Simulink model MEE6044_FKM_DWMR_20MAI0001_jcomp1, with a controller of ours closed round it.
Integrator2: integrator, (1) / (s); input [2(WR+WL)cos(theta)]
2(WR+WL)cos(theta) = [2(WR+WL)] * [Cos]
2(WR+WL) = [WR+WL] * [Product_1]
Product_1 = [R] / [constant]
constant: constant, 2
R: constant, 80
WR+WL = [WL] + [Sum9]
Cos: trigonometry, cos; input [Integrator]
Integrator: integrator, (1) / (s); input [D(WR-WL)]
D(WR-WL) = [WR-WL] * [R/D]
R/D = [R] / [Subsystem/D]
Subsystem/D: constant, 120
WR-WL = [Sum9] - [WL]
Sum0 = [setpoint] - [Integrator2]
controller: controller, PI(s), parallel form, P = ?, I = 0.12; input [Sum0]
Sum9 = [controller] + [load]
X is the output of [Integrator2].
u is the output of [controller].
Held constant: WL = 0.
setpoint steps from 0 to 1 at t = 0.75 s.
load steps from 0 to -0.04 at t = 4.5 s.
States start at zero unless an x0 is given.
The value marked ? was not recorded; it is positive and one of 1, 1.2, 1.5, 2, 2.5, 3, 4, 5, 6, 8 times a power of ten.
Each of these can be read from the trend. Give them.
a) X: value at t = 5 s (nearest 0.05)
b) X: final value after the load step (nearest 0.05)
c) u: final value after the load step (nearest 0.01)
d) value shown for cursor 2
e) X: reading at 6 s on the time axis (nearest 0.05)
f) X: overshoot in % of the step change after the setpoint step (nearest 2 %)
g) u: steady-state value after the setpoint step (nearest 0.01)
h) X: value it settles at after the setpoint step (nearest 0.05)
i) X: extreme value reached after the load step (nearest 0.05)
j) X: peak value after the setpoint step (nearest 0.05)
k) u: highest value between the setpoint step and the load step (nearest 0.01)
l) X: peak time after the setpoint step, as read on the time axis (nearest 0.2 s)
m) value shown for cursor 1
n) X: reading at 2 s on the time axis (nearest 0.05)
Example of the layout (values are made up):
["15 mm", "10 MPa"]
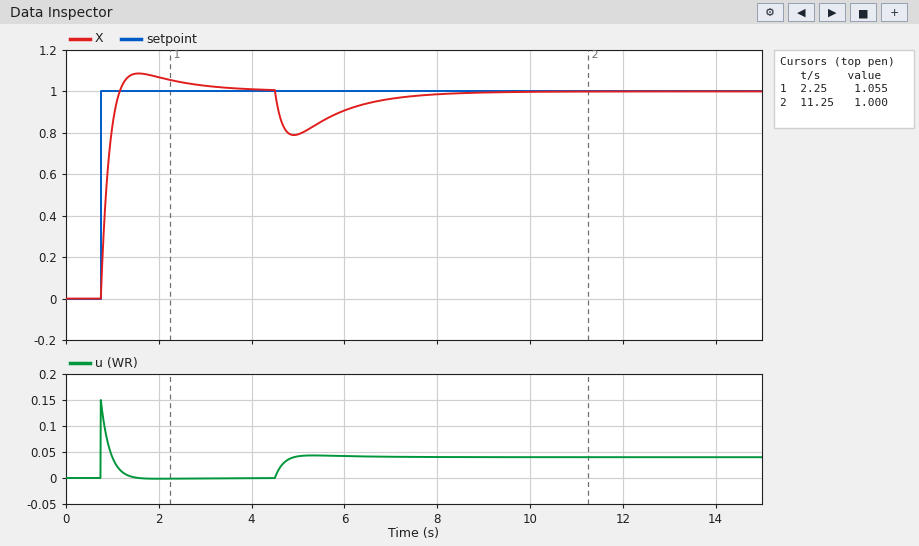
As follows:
["0.80", "1.00", "0.04", "1.000", "0.90", "8 %", "0.00", "1.00", "0.80", "1.10", "0.15", "1.6 s", "1.055", "1.05"]
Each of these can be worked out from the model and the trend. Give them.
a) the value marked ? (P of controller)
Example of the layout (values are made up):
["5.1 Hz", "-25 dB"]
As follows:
["0.15"]
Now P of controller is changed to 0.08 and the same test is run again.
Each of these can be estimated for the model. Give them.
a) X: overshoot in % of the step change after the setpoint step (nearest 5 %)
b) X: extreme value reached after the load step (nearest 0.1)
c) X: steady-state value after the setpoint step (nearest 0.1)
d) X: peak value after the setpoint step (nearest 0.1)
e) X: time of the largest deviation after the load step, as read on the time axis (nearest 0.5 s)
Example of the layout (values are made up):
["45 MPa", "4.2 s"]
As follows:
["20 %", "0.7", "1.0", "1.2", "5.0 s"]
